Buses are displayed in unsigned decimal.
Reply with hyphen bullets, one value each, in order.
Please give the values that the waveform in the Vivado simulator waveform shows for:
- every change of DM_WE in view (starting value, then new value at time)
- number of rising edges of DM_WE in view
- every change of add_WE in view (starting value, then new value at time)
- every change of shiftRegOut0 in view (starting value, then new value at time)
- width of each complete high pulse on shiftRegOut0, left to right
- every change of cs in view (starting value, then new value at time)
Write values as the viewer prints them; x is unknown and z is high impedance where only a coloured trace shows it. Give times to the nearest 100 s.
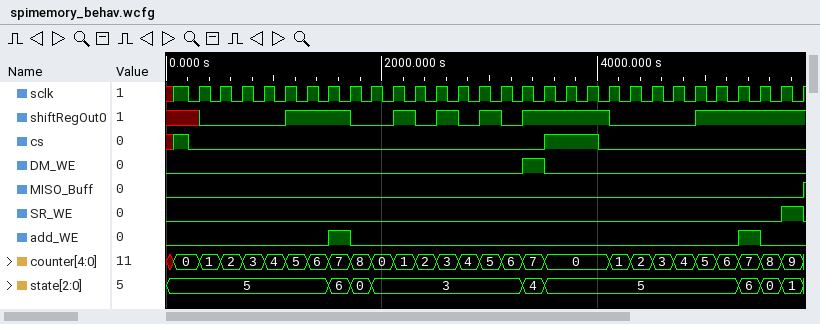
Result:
- 0, 1 at 3300 s, 0 at 3500 s
- 1
- 0, 1 at 1500 s, 0 at 1700 s, 1 at 5300 s, 0 at 5500 s
- x, 0 at 300 s, 1 at 1100 s, 0 at 1700 s, 1 at 2100 s, 0 at 2300 s, 1 at 2500 s, 0 at 2700 s, 1 at 2900 s, 0 at 3100 s, 1 at 3300 s, 0 at 4100 s, 1 at 4900 s
- 600 s, 200 s, 200 s, 200 s, 800 s
- x, 1 at 100 s, 0 at 200 s, 1 at 3500 s, 0 at 4000 s
